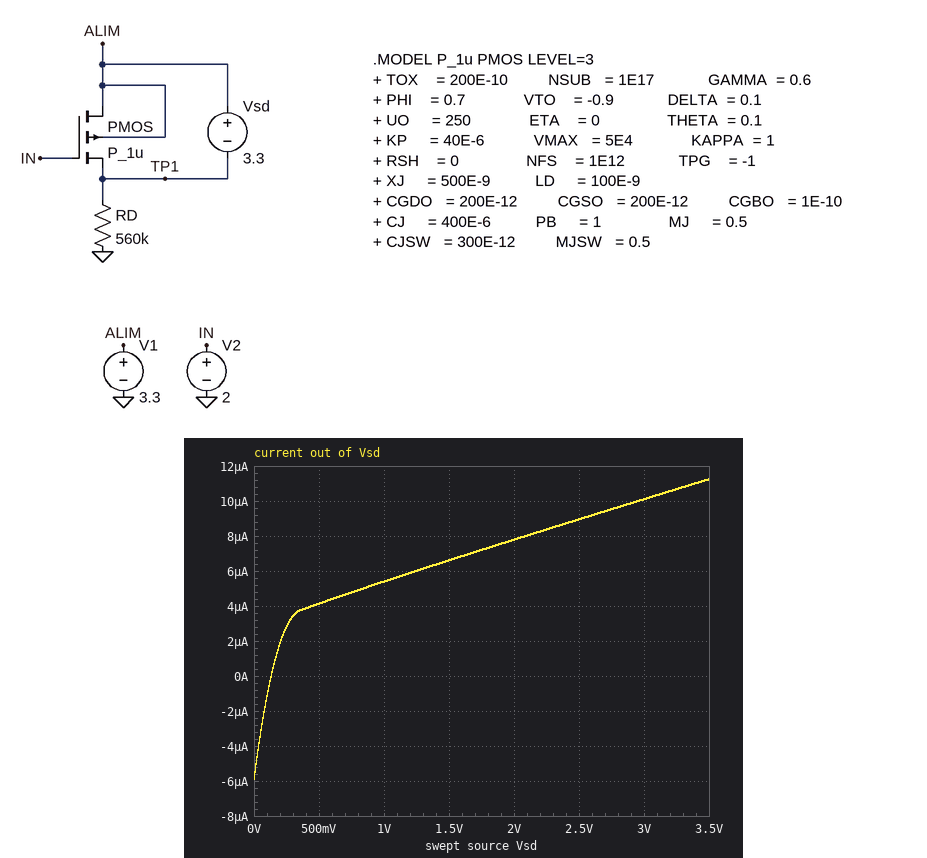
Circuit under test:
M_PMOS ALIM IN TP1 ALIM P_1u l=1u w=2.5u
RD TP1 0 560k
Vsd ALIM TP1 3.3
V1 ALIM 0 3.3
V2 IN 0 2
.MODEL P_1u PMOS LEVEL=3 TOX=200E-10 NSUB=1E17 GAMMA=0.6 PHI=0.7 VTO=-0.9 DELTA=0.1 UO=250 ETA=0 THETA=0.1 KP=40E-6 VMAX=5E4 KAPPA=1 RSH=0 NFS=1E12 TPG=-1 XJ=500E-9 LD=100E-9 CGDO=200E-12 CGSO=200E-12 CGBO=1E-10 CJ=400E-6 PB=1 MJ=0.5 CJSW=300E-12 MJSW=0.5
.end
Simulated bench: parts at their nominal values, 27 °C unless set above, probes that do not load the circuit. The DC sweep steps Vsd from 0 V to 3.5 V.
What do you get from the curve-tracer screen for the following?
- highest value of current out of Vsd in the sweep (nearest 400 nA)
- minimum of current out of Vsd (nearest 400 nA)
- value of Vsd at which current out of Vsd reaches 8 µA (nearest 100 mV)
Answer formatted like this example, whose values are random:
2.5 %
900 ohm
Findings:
11.2 µA
-6.0 µA
2.1 V
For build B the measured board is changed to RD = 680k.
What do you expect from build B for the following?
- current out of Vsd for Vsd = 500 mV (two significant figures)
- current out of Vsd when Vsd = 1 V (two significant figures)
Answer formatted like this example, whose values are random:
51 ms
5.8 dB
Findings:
5.0 µA
6.1 µA
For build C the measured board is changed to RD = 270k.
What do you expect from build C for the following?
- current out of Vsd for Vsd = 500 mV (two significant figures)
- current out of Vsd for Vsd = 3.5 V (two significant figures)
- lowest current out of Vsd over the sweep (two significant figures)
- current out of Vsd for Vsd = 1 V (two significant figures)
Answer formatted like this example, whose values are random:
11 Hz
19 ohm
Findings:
-1.2 µA
12 µA
-12 µA
990 nA
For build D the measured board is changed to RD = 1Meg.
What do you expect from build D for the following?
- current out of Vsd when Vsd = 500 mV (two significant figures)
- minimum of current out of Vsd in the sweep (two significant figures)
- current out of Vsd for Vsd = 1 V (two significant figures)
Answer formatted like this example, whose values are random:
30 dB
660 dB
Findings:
6.3 µA
-3.3 µA
7.2 µA
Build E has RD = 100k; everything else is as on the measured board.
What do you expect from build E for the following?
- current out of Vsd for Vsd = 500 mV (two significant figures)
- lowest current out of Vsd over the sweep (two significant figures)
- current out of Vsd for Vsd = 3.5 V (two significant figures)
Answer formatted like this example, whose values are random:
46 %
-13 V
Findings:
-19 µA
-33 µA
13 µA
